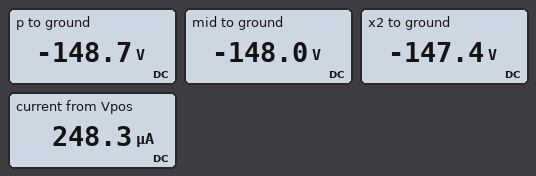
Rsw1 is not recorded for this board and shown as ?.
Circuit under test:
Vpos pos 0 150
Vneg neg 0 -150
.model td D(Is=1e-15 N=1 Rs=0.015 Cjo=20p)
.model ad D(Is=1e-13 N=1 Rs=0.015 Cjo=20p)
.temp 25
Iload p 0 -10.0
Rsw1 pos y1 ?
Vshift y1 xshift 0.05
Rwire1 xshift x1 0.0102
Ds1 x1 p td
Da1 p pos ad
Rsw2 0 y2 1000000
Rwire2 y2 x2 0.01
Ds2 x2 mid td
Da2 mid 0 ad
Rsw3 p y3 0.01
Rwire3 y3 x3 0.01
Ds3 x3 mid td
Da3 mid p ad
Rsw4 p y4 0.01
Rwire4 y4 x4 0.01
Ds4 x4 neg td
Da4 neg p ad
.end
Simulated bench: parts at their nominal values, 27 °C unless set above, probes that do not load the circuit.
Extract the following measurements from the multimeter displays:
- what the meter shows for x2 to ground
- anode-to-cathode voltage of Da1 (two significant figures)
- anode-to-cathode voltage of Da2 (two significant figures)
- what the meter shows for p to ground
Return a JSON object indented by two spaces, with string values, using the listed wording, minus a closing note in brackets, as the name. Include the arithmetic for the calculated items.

{
  "what the meter shows for x2 to ground": "-147.4 V",
  "anode-to-cathode voltage of Da1": "-148.7 V - 150 V = -300 V",
  "anode-to-cathode voltage of Da2": "-148 V = -150 V",
  "what the meter shows for p to ground": "-148.7 V"
}
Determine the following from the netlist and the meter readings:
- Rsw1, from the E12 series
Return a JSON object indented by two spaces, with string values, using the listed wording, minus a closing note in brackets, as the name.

{
  "Rsw1, from the E12 series": "1.2 MΩ"
}
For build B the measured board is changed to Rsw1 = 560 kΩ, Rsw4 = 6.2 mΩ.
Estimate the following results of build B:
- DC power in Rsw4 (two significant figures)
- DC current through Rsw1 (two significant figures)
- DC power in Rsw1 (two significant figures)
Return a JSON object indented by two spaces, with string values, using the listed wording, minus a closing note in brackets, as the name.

{
  "DC power in Rsw4": "620 mW",
  "DC current through Rsw1": "530 µA",
  "DC power in Rsw1": "160 mW"
}
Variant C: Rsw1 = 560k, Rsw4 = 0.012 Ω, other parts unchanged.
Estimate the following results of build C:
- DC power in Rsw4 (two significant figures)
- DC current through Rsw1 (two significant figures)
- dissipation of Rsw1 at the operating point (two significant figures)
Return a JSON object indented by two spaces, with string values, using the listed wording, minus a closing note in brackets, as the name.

{
  "DC power in Rsw4": "1.2 W",
  "DC current through Rsw1": "530 µA",
  "dissipation of Rsw1 at the operating point": "160 mW"
}
